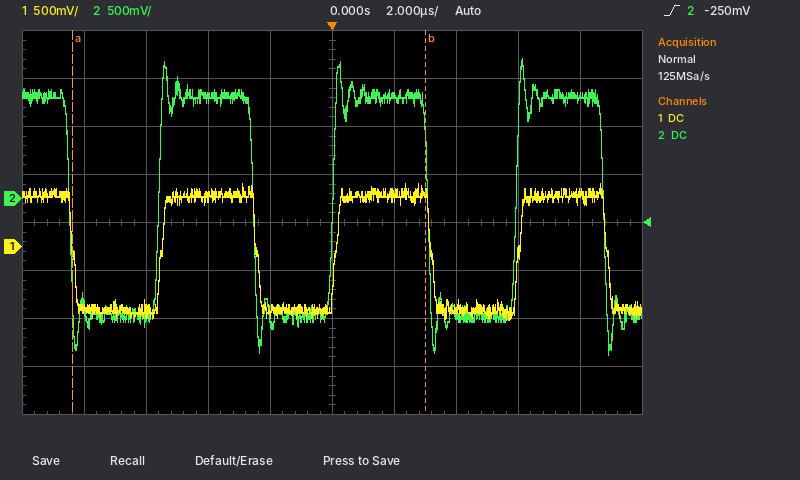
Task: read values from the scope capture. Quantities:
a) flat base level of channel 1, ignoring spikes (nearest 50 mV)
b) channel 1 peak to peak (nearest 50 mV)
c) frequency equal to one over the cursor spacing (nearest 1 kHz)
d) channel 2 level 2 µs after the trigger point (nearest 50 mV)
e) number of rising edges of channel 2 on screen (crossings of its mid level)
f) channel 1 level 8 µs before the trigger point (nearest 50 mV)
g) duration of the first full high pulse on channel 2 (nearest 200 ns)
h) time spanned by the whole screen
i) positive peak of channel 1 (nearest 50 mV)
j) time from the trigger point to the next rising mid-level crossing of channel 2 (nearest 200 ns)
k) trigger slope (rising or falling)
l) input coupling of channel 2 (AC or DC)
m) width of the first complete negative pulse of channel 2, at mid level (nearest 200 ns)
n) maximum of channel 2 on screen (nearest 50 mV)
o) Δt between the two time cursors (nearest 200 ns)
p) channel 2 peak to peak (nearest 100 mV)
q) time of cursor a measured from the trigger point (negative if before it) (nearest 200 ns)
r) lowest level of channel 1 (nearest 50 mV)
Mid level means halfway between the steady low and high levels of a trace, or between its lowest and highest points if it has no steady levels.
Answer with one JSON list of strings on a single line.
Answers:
["-650 mV", "1.40 V", "88 kHz", "1.05 V", "3", "-650 mV", "3.0 µs", "20 µs", "650 mV", "6.0 µs", "rising", "DC", "2.8 µs", "1.45 V", "11.4 µs", "3.10 V", "-8.4 µs", "-750 mV"]
